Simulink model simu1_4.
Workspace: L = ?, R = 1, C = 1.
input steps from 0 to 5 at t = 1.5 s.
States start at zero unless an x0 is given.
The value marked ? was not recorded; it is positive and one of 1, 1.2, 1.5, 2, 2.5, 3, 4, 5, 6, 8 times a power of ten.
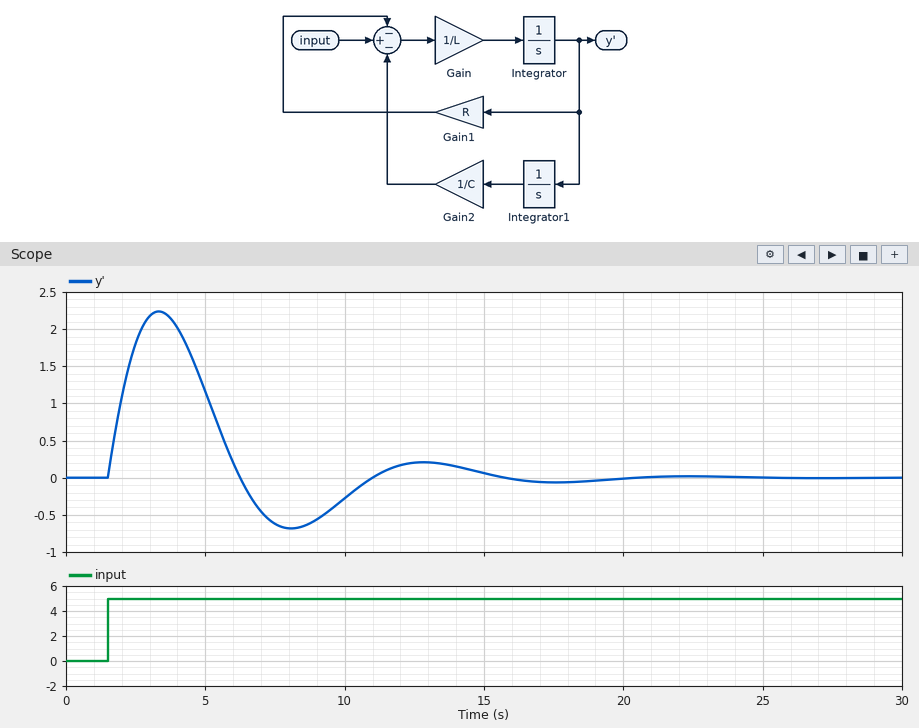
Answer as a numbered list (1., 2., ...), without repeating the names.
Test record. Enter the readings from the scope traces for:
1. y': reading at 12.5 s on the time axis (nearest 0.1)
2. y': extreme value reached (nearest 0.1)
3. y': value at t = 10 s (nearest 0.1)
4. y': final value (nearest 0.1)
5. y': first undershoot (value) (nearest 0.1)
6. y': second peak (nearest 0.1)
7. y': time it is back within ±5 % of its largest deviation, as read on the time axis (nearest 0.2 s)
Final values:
1. 0.2
2. 2.2
3. -0.3
4. 0.0
5. -0.7
6. 0.2
7. 14.4 s
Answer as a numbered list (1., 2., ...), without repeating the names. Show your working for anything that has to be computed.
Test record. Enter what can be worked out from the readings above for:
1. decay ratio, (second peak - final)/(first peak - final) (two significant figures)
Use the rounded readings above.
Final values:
1. (0.2 - 0) / (2.2 - 0) = 0.091
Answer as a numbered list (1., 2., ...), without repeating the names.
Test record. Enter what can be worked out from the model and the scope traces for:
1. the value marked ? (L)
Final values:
1. 2
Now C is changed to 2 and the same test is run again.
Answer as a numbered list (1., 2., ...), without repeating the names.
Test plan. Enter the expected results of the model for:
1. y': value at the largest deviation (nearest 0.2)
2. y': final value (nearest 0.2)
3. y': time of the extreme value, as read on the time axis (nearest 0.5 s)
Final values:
1. 2.8
2. 0.0
3. 4.0 s
